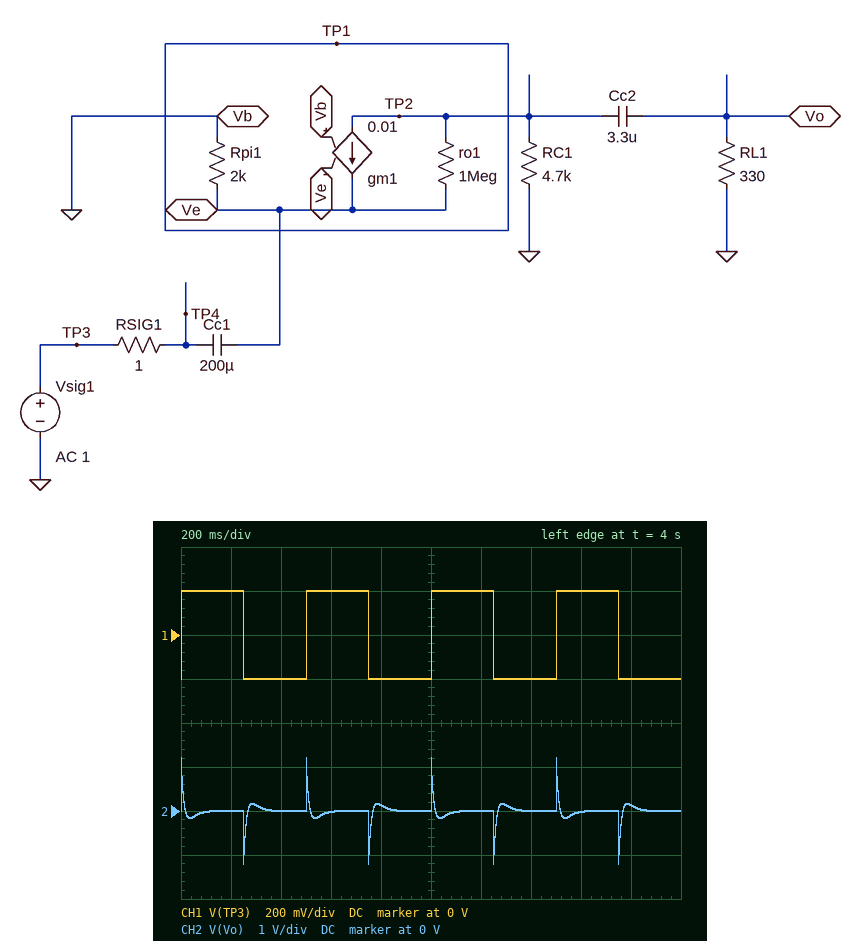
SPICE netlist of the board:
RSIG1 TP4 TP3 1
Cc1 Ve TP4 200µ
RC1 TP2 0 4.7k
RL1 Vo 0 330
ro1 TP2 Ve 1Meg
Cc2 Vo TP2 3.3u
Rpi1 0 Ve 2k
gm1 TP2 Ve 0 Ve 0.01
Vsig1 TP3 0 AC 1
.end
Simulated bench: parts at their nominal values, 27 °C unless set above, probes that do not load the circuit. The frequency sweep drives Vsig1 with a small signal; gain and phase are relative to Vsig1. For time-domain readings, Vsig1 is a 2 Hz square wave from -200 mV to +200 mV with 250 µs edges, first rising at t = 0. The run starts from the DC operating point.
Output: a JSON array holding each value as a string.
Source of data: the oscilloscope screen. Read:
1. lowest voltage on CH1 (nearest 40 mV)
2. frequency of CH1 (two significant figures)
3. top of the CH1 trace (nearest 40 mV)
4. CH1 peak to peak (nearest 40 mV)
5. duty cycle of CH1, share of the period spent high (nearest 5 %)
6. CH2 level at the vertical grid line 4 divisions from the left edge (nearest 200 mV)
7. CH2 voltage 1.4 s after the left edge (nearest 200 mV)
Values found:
["-200 mV", "2.0 Hz", "200 mV", "400 mV", "50 %", "200 mV", "0 V"]
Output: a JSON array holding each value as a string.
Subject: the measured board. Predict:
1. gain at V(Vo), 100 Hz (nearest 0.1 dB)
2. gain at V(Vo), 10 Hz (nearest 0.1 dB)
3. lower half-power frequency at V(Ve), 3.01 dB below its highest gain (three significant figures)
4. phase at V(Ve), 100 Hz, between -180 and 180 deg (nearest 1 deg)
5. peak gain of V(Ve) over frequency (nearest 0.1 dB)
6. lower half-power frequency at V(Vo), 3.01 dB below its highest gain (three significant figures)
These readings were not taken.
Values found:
["9.6 dB", "4.6 dB", "8.26 Hz", "5 deg", "-0.1 dB", "13.9 Hz"]
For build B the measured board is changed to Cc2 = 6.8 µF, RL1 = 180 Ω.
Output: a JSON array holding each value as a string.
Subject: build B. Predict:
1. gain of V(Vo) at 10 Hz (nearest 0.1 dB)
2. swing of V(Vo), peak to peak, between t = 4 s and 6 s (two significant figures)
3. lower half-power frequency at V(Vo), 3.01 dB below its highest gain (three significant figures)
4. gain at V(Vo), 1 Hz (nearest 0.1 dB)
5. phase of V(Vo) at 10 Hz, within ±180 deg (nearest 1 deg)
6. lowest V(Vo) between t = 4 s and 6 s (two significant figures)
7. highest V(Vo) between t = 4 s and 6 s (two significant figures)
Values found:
["1.5 dB", "1.4 V", "10.3 Hz", "-27.5 dB", "65 deg", "-680 mV", "680 mV"]
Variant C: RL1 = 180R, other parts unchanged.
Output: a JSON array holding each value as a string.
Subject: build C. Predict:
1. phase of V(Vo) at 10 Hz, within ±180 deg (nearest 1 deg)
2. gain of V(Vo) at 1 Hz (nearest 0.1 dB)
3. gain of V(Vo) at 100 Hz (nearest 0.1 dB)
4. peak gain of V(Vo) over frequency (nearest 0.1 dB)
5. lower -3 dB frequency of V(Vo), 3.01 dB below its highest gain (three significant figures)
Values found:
["84 deg", "-33.7 dB", "4.6 dB", "4.7 dB", "14.2 Hz"]
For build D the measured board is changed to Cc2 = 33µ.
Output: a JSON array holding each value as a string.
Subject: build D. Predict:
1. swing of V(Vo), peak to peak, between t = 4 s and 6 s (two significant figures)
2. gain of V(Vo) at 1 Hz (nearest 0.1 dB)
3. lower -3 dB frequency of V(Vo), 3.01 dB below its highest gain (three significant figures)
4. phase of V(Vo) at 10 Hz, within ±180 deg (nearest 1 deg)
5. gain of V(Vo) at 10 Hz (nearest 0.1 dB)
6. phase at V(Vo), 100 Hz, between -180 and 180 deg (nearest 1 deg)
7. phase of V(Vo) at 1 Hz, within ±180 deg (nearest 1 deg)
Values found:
["2.5 V", "-11.6 dB", "8.38 Hz", "45 deg", "7.4 dB", "5 deg", "127 deg"]
